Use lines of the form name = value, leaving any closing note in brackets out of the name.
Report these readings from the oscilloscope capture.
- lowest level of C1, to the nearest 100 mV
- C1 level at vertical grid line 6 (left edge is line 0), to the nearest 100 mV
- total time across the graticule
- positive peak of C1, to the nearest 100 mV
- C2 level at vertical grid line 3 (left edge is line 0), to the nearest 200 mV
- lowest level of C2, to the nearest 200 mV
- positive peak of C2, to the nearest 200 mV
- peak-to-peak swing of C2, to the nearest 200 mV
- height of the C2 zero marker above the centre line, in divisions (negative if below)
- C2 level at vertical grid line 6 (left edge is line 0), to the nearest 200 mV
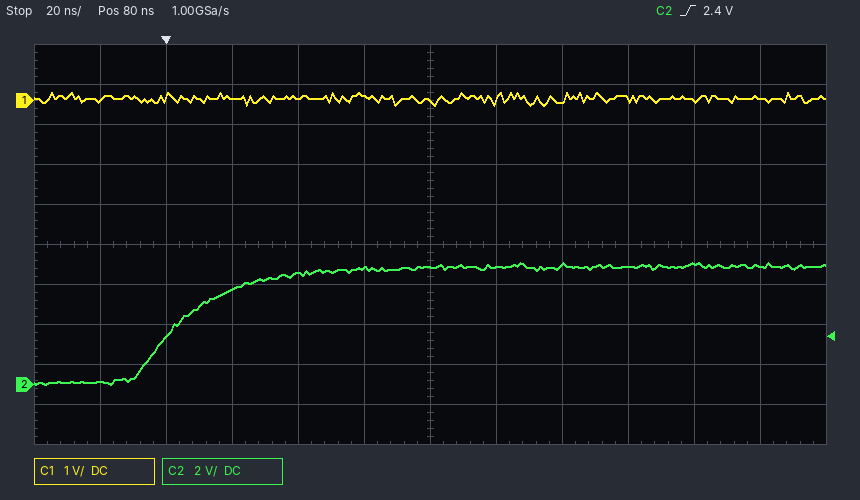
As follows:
lowest level of C1, to the nearest 100 mV = -100 mV
C1 level at vertical grid line 6 (left edge is line 0), to the nearest 100 mV = 0.0 V
total time across the graticule = 240 ns
positive peak of C1, to the nearest 100 mV = 200 mV
C2 level at vertical grid line 3 (left edge is line 0), to the nearest 200 mV = 4.8 V
lowest level of C2, to the nearest 200 mV = 0.0 V
positive peak of C2, to the nearest 200 mV = 6.0 V
peak-to-peak swing of C2, to the nearest 200 mV = 6.0 V
height of the C2 zero marker above the centre line, in divisions = -3.5 div
C2 level at vertical grid line 6 (left edge is line 0), to the nearest 200 mV = 5.8 V
